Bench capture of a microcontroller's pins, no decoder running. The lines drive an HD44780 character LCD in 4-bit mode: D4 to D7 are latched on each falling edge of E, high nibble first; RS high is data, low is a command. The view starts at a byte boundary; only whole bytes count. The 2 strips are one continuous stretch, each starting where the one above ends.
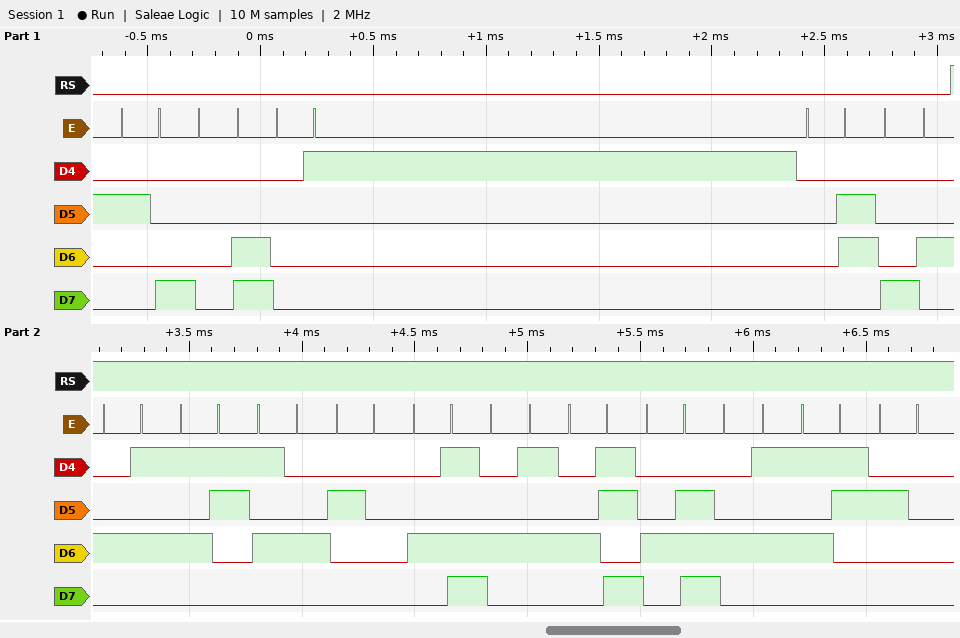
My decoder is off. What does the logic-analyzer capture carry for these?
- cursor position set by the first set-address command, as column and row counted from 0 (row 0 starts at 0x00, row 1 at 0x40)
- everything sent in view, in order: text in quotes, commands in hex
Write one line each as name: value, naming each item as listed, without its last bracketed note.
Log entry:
cursor position set by the first set-address command, as column and row counted from 0: column 4, row 0
everything sent in view, in order: text in quotes, commands in hex: 0x28 0x0C 0x01 0x06 0x84 "EST MEKNES "
